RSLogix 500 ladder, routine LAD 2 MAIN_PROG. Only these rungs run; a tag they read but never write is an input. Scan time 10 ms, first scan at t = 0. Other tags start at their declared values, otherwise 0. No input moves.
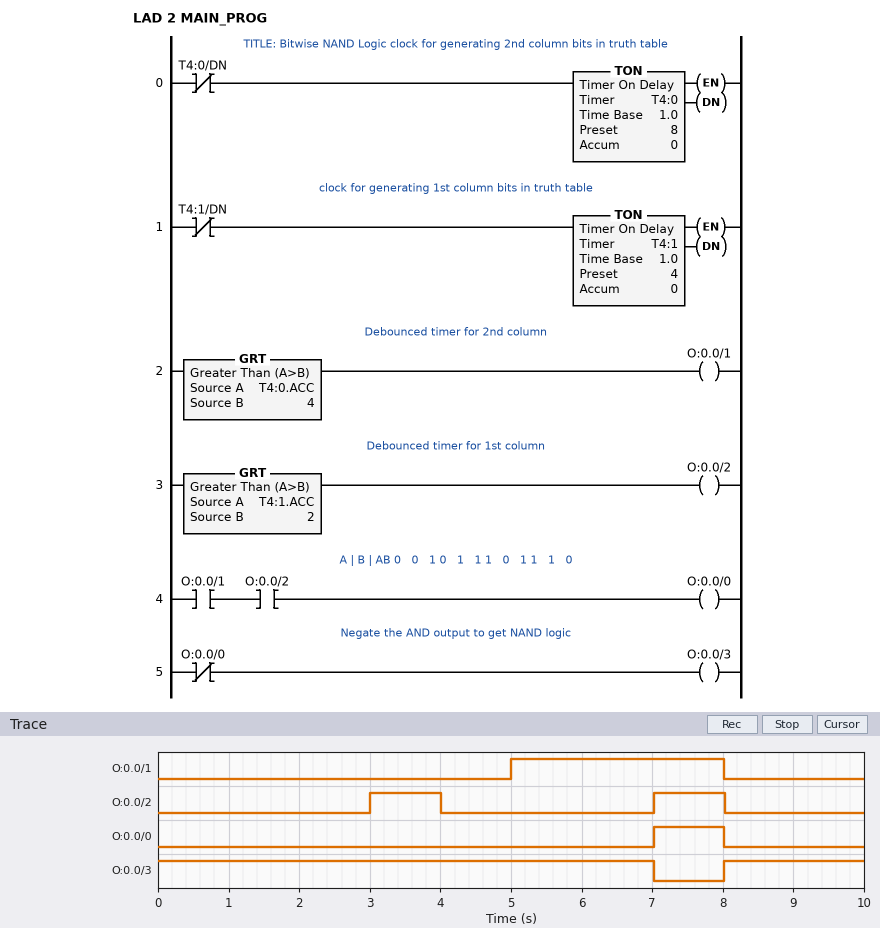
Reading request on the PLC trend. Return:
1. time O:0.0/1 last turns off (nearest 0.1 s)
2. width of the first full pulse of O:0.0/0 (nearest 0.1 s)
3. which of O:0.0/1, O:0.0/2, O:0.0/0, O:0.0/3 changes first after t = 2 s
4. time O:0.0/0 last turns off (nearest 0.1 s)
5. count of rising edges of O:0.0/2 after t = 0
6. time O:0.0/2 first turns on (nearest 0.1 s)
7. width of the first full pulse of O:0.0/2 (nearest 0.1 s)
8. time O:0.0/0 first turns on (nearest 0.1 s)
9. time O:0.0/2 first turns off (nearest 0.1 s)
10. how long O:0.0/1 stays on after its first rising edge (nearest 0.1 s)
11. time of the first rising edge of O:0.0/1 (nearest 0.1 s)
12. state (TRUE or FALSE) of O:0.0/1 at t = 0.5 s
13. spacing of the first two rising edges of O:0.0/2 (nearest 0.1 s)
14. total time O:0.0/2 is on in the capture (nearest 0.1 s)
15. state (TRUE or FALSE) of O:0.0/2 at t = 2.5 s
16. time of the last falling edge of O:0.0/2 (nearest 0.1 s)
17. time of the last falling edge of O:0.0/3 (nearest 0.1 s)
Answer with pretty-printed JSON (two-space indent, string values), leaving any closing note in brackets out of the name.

{
  "time O:0.0/1 last turns off": "8.0 s",
  "width of the first full pulse of O:0.0/0": "1.0 s",
  "which of O:0.0/1, O:0.0/2, O:0.0/0, O:0.0/3 changes first after t = 2 s": "O:0.0/2",
  "time O:0.0/0 last turns off": "8.0 s",
  "count of rising edges of O:0.0/2 after t = 0": "2",
  "time O:0.0/2 first turns on": "3.0 s",
  "width of the first full pulse of O:0.0/2": "1.0 s",
  "time O:0.0/0 first turns on": "7.0 s",
  "time O:0.0/2 first turns off": "4.0 s",
  "how long O:0.0/1 stays on after its first rising edge": "3.0 s",
  "time of the first rising edge of O:0.0/1": "5.0 s",
  "state (TRUE or FALSE) of O:0.0/1 at t = 0.5 s": "FALSE",
  "spacing of the first two rising edges of O:0.0/2": "4.0 s",
  "total time O:0.0/2 is on in the capture": "2.0 s",
  "state (TRUE or FALSE) of O:0.0/2 at t = 2.5 s": "FALSE",
  "time of the last falling edge of O:0.0/2": "8.0 s",
  "time of the last falling edge of O:0.0/3": "7.0 s"
}
